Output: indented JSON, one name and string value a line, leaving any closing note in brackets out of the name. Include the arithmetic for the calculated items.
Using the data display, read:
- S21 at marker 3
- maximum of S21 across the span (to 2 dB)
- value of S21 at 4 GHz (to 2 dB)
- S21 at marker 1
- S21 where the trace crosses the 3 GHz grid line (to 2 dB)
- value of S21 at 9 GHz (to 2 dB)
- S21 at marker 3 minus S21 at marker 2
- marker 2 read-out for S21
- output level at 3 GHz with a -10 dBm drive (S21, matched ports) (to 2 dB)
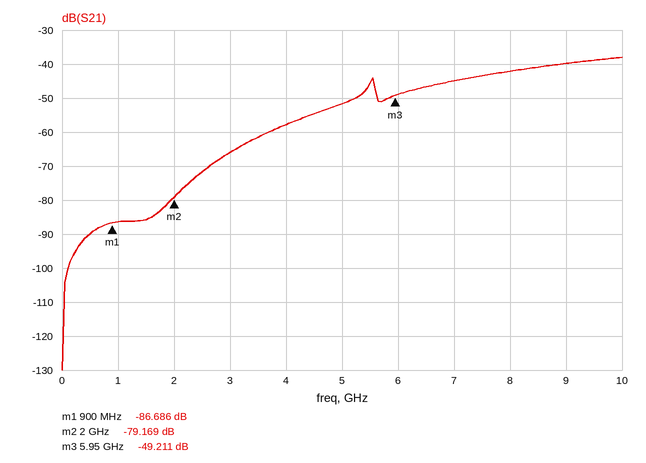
{
  "S21 at marker 3": "-49.211 dB",
  "maximum of S21 across the span": "-38 dB",
  "value of S21 at 4 GHz": "-58 dB",
  "S21 at marker 1": "-86.686 dB",
  "S21 where the trace crosses the 3 GHz grid line": "-66 dB",
  "value of S21 at 9 GHz": "-40 dB",
  "S21 at marker 3 minus S21 at marker 2": "-49.211 − (-79.169) = 29.958 dB",
  "marker 2 read-out for S21": "-79.169 dB",
  "output level at 3 GHz with a -10 dBm drive (S21, matched ports)": "-10 dBm + (-66 dB) = -76 dBm"
}
